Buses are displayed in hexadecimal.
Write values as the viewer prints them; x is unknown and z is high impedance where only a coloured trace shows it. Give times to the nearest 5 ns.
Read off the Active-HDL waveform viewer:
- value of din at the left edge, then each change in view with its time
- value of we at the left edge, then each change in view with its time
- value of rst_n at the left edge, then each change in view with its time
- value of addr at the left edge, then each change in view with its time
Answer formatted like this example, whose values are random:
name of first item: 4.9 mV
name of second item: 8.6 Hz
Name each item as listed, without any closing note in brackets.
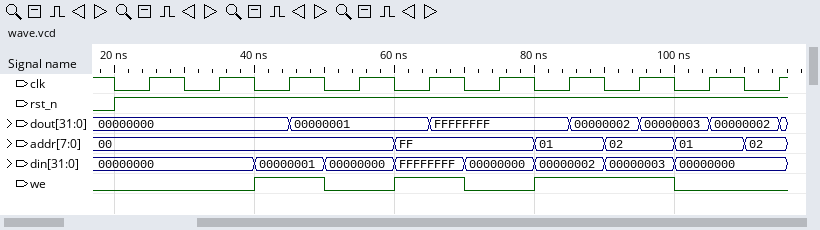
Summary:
value of din at the left edge, then each change in view with its time: 00000000, 00000001 at 40 ns, 00000000 at 50 ns, FFFFFFFF at 60 ns, 00000000 at 70 ns, 00000002 at 80 ns, 00000003 at 90 ns, 00000000 at 100 ns
value of we at the left edge, then each change in view with its time: 0, 1 at 40 ns, 0 at 50 ns, 1 at 60 ns, 0 at 70 ns, 1 at 80 ns, 0 at 100 ns
value of rst_n at the left edge, then each change in view with its time: 0, 1 at 20 ns
value of addr at the left edge, then each change in view with its time: 00, FF at 60 ns, 01 at 80 ns, 02 at 90 ns, 01 at 100 ns, 02 at 110 ns
